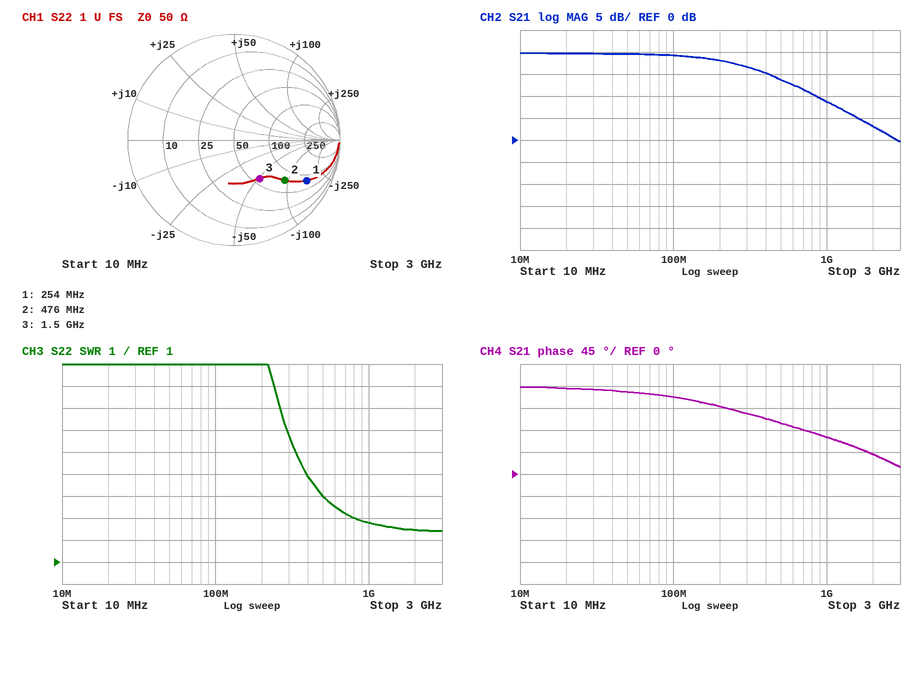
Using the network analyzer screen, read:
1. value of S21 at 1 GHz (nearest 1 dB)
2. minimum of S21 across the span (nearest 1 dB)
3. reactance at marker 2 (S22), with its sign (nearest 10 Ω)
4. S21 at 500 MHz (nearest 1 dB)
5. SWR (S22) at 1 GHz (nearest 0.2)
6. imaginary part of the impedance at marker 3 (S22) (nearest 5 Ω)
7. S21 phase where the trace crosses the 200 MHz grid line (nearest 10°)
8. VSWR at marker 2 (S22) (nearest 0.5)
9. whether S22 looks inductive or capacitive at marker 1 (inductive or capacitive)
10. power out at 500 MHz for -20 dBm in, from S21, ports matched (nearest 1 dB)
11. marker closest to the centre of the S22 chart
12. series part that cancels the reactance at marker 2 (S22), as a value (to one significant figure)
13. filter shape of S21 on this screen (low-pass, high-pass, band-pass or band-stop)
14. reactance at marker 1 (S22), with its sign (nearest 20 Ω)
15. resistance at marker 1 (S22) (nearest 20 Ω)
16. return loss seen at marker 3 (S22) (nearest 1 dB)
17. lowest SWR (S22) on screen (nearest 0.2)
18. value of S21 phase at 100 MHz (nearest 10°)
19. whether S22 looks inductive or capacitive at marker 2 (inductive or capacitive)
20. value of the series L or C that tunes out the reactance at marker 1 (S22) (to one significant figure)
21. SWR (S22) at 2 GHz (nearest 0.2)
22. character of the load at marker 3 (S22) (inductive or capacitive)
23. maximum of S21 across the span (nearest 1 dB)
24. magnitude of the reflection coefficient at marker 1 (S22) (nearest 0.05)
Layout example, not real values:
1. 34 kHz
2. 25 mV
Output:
1. 9 dB
2. 0 dB
3. -90 Ω
4. 14 dB
5. 2.8
6. -50 Ω
7. 140°
8. 4.0
9. capacitive
10. -6 dBm
11. marker 3
12. 30 nH
13. low-pass
14. -160 Ω
15. 80 Ω
16. 7 dB
17. 2.4
18. 160°
19. capacitive
20. 100 nH
21. 2.4
22. capacitive
23. 20 dB
24. 0.80
